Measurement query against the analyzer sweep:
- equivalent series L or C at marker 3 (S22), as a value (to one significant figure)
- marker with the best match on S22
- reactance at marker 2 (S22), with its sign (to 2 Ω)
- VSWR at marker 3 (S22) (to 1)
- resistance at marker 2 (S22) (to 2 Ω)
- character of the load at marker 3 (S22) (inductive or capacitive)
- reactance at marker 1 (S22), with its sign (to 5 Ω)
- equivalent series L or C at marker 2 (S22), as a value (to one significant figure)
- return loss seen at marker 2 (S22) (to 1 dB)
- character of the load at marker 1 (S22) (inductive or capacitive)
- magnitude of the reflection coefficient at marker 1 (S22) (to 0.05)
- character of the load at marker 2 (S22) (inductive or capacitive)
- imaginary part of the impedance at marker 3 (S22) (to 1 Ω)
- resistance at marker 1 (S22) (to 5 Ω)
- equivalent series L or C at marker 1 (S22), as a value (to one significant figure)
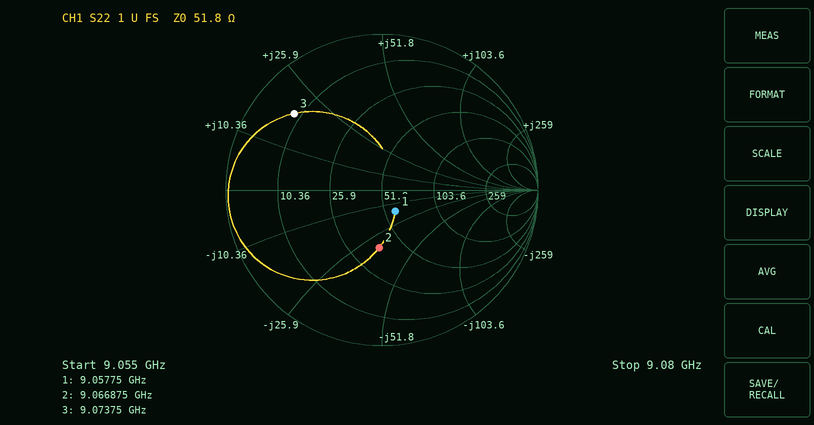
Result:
300 pH
marker 1
-32 Ω
7
38 Ω
inductive
-15 Ω
500 fF
9 dB
capacitive
0.15
capacitive
+19 Ω
60 Ω
1 pF
